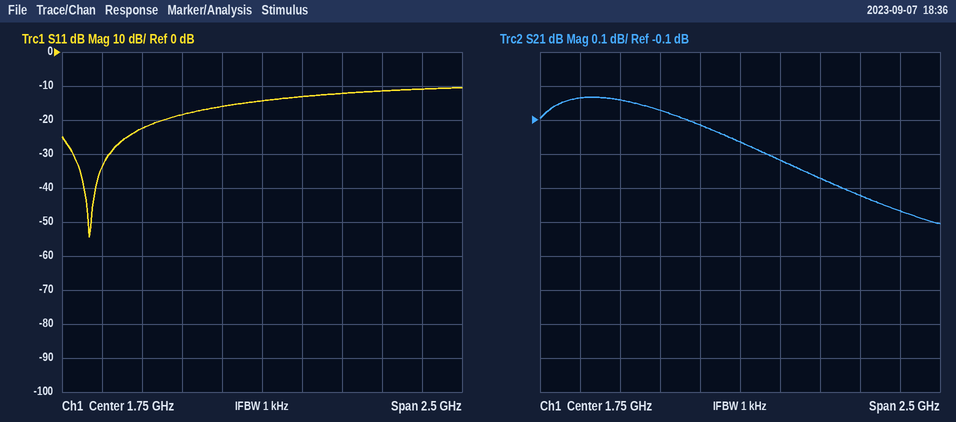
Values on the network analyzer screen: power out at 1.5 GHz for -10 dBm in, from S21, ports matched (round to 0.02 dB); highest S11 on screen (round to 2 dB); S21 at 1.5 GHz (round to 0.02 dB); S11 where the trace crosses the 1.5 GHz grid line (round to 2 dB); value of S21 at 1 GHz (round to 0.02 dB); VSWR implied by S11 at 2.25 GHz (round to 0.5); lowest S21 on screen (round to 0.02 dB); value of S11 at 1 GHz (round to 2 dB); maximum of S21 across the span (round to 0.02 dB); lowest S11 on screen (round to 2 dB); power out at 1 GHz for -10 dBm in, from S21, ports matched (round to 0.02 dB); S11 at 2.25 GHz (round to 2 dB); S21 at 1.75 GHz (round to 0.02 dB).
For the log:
-10.12 dBm
-10 dB
-0.12 dB
-16 dB
-0.04 dB
1.5
-0.40 dB
-22 dB
-0.04 dB
-54 dB
-10.04 dBm
-12 dB
-0.16 dB
